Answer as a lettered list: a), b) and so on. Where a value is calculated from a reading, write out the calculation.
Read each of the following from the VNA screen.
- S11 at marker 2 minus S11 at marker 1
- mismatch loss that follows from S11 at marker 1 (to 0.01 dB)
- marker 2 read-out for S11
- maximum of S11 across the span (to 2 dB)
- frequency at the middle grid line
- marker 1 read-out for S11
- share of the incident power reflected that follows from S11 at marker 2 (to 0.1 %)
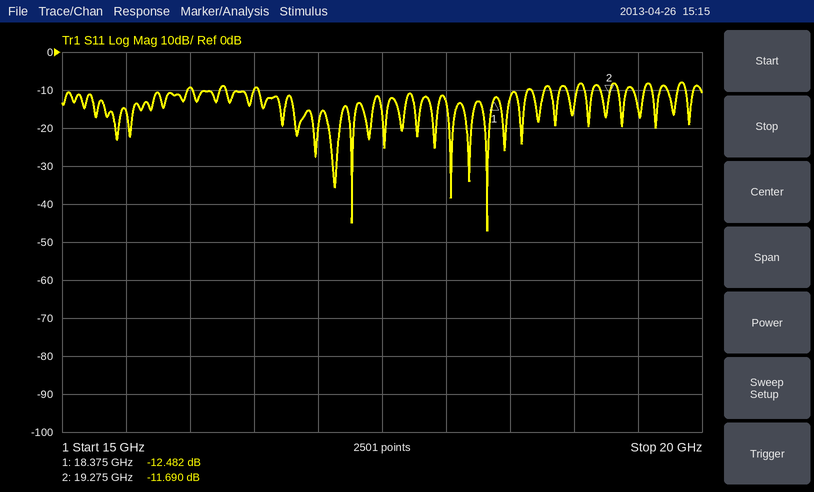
a) -11.69 − (-12.482) = 0.792 dB
b) −10 log10(1 − 10^(-12.482/10)) ≈ 0.25 dB
c) -11.690 dB
d) -8 dB
e) 17.5 GHz
f) -12.482 dB
g) 10^(-11.69/10) ≈ 6.8 %
